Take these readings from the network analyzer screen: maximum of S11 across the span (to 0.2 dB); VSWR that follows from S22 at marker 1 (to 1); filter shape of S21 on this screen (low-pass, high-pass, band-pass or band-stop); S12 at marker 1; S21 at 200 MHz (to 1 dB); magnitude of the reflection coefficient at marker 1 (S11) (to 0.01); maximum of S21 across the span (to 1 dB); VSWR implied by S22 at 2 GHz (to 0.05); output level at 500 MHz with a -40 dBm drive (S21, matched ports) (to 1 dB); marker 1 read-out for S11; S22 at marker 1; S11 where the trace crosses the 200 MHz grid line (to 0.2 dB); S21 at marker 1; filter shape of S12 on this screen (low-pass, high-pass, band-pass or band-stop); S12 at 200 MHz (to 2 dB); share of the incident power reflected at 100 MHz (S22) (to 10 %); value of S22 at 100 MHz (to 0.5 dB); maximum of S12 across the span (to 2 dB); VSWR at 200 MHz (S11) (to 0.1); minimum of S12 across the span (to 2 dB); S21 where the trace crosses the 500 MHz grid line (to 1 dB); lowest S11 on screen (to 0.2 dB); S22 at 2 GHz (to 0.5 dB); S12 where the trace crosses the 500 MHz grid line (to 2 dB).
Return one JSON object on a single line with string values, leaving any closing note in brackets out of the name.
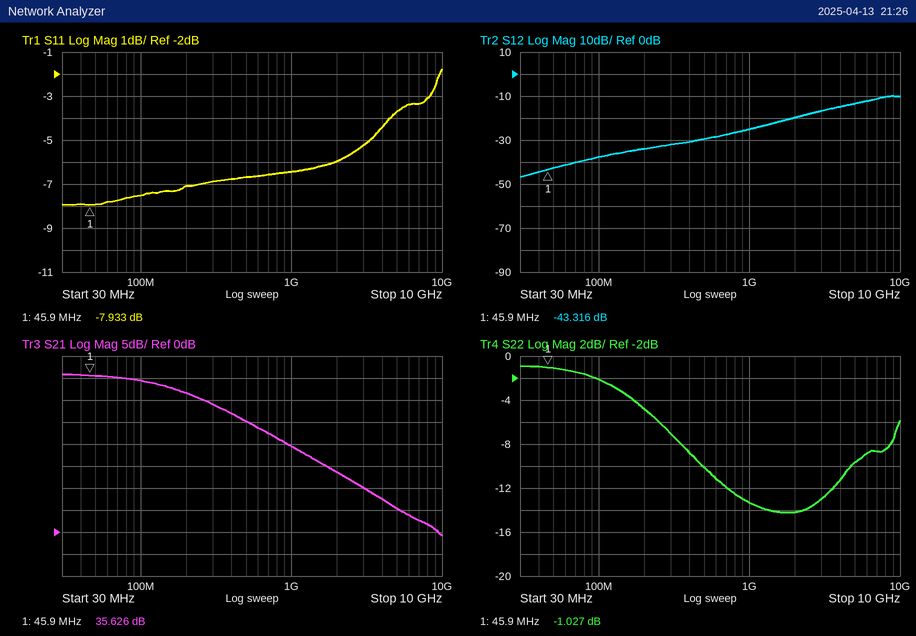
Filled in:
{"maximum of S11 across the span": "-1.8 dB", "VSWR that follows from S22 at marker 1": "17", "filter shape of S21 on this screen": "low-pass", "S12 at marker 1": "-43.316 dB", "S21 at 200 MHz": "32 dB", "magnitude of the reflection coefficient at marker 1 (S11)": "0.40", "maximum of S21 across the span": "36 dB", "VSWR implied by S22 at 2 GHz": "1.50", "output level at 500 MHz with a -40 dBm drive (S21, matched ports)": "-15 dBm", "marker 1 read-out for S11": "-7.933 dB", "S22 at marker 1": "-1.027 dB", "S11 where the trace crosses the 200 MHz grid line": "-7.0 dB", "S21 at marker 1": "35.626 dB", "filter shape of S12 on this screen": "high-pass", "S12 at 200 MHz": "-34 dB", "share of the incident power reflected at 100 MHz (S22)": "60 %", "value of S22 at 100 MHz": "-2.0 dB", "maximum of S12 across the span": "-10 dB", "VSWR at 200 MHz (S11)": "2.6", "minimum of S12 across the span": "-46 dB", "S21 where the trace crosses the 500 MHz grid line": "25 dB", "lowest S11 on screen": "-8.0 dB", "S22 at 2 GHz": "-14.0 dB", "S12 where the trace crosses the 500 MHz grid line": "-30 dB"}
